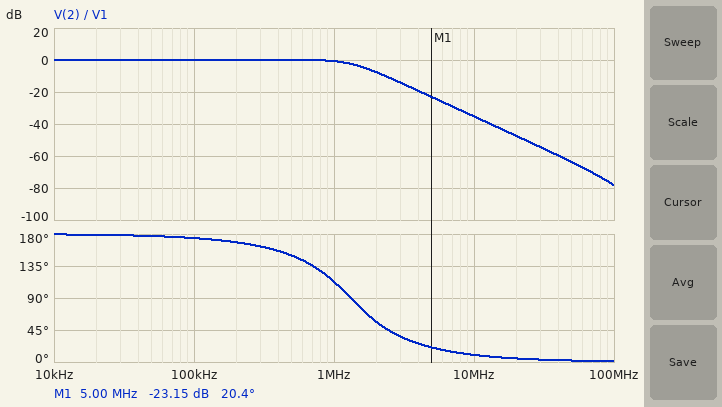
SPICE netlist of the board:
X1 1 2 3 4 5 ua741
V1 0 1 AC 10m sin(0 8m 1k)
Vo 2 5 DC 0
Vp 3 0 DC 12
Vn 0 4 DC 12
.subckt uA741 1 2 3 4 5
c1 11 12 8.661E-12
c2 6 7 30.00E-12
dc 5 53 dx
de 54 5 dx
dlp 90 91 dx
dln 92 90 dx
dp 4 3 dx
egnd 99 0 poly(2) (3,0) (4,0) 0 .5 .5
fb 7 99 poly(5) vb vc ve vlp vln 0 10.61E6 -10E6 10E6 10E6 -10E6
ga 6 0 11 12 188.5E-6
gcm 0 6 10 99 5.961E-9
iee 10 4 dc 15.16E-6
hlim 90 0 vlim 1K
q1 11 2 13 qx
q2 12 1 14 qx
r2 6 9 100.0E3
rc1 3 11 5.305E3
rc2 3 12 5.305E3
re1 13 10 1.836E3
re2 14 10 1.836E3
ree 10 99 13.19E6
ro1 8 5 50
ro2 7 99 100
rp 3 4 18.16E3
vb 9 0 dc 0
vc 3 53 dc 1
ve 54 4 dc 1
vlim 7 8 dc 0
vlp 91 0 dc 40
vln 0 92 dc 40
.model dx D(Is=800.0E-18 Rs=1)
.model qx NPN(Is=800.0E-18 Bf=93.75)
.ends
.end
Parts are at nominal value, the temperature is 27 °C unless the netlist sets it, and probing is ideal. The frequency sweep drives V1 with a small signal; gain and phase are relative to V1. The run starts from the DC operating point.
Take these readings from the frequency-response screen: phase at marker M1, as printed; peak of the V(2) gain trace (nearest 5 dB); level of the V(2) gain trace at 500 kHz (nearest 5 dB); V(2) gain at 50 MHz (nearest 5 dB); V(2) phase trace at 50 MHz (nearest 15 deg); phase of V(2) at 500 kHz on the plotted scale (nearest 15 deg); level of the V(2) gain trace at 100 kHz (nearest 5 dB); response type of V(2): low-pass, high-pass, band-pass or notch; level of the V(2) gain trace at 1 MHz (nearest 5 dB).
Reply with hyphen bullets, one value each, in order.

- 20.4 deg
- 0 dB
- 0 dB
- -65 dB
- 0 deg
- 150 deg
- 0 dB
- low-pass
- 0 dB
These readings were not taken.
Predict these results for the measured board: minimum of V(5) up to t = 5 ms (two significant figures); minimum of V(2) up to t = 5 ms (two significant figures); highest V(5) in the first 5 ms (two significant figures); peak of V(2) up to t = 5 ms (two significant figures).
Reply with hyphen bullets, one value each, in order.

- -8.0 mV
- -8.0 mV
- 8.0 mV
- 8.0 mV
